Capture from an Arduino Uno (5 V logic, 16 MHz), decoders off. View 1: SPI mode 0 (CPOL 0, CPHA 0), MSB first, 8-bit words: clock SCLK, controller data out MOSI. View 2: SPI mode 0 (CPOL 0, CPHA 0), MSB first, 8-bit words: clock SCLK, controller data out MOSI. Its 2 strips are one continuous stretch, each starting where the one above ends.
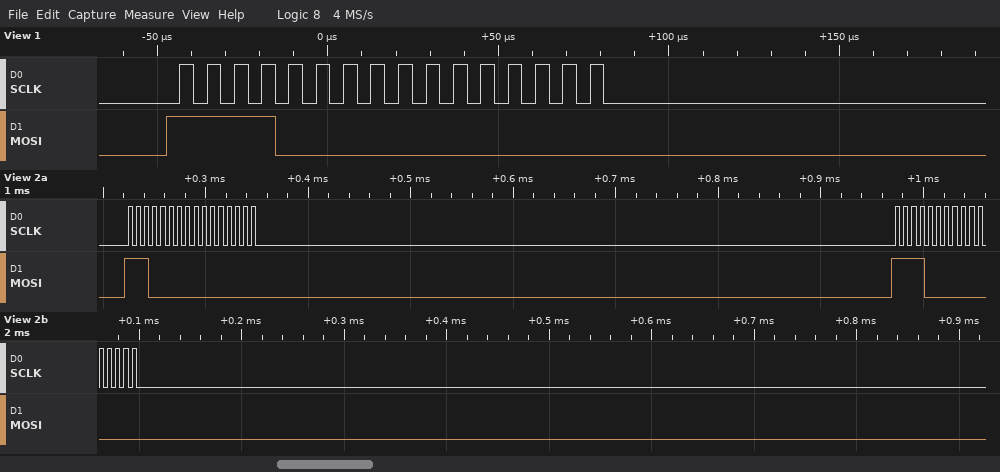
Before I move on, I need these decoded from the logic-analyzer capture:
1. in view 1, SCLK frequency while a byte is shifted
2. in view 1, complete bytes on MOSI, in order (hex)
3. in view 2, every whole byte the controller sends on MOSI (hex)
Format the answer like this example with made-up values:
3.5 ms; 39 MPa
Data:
125 kHz; F0 00; E0 00 F0 00
